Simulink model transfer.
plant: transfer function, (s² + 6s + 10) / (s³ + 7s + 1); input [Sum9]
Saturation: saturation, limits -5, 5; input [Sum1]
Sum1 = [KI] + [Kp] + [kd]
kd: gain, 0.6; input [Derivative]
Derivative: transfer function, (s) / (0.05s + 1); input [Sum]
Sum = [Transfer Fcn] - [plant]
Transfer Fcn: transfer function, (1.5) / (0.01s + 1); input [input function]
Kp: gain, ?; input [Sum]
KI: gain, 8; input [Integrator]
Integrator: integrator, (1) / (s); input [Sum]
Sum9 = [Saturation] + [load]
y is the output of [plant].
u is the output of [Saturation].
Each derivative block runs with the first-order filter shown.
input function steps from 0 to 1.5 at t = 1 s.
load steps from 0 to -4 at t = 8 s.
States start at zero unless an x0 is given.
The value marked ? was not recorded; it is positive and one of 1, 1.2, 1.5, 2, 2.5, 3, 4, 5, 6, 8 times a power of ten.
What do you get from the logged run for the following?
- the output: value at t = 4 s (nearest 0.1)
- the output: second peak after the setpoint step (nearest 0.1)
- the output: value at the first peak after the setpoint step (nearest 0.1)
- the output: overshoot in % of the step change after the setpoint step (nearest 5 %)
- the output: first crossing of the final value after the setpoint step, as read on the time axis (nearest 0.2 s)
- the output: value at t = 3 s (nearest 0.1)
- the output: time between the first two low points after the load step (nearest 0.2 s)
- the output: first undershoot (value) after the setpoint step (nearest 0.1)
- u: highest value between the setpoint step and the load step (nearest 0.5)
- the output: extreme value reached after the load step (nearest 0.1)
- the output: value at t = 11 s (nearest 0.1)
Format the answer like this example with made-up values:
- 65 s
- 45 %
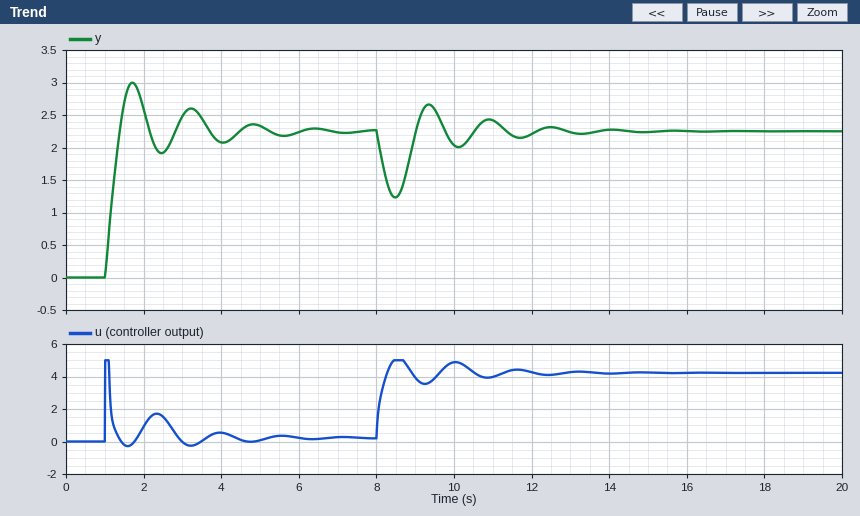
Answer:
- 2.1
- 2.6
- 3.0
- 35 %
- 1.4 s
- 2.5
- 1.6 s
- 1.9
- 5.0
- 1.2
- 2.4
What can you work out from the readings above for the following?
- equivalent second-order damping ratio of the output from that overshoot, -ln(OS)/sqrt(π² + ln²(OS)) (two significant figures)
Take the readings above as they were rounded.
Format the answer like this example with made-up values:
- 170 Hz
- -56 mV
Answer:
- 0.32
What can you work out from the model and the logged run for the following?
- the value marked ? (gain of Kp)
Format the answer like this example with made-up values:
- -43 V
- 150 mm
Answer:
- 2
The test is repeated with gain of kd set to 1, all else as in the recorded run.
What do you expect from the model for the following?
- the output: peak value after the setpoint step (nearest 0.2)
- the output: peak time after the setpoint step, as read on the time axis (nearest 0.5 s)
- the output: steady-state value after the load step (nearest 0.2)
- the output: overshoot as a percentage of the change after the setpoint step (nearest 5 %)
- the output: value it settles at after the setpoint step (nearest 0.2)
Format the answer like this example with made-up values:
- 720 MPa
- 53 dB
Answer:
- 2.8
- 2.0 s
- 2.2
- 25 %
- 2.2
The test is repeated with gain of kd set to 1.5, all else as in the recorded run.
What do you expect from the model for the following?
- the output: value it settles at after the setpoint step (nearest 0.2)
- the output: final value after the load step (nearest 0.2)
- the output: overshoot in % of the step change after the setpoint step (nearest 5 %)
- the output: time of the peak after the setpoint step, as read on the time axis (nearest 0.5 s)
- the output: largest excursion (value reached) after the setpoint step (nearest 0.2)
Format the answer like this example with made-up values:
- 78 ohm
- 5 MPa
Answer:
- 2.2
- 2.2
- 25 %
- 2.0 s
- 2.8
